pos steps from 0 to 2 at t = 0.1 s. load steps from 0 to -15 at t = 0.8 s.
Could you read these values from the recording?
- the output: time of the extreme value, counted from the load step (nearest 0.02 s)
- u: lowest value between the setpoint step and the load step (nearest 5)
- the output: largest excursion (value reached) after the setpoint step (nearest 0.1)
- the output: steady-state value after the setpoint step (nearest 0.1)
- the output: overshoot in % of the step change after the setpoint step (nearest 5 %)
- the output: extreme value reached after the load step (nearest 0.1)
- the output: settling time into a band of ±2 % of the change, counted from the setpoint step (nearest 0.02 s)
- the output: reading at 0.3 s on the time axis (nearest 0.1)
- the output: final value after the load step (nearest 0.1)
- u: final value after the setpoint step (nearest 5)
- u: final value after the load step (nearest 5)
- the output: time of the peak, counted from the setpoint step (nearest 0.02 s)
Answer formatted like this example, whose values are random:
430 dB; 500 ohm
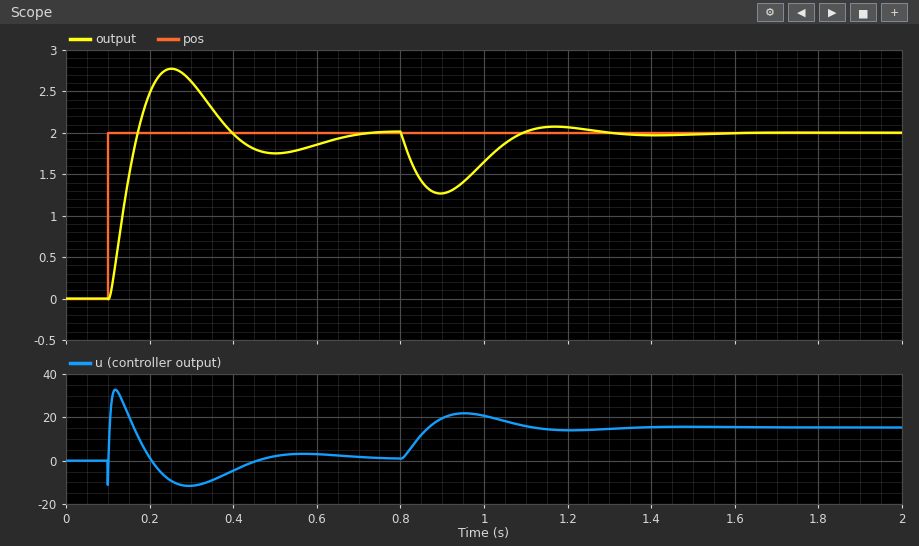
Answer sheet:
0.10 s; -10; 2.8; 2.0; 40 %; 1.3; 0.58 s; 2.6; 2.0; 0; 15; 0.16 s
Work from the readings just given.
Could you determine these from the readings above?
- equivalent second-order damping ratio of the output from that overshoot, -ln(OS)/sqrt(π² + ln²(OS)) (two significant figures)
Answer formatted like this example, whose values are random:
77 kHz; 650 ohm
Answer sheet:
0.28
